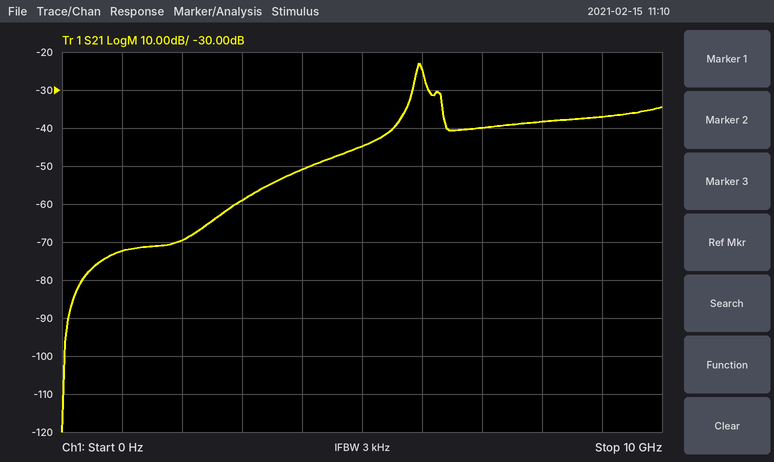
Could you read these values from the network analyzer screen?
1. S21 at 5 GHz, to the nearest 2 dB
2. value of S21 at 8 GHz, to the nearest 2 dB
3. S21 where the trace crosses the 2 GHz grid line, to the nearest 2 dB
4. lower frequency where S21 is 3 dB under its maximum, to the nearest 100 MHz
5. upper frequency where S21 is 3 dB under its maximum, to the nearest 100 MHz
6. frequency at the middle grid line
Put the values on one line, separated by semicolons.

-44 dB; -38 dB; -70 dB; 5.9 GHz; 6.0 GHz; 5 GHz
